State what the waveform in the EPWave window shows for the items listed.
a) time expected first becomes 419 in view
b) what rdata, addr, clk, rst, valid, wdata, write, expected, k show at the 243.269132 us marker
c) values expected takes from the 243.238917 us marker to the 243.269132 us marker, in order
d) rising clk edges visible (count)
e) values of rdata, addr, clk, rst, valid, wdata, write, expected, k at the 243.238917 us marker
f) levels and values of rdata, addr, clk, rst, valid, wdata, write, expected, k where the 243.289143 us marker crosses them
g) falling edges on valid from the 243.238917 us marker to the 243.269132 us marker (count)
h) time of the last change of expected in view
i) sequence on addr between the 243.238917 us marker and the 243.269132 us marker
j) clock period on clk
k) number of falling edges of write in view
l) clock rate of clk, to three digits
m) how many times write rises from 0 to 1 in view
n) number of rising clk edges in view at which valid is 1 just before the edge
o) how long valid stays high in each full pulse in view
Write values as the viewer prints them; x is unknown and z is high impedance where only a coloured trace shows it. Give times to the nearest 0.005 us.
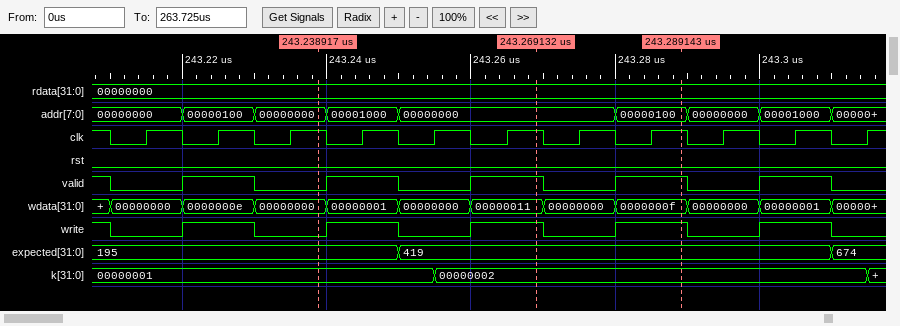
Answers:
243.25 us
rdata=00000000, addr=00000000, clk=1, rst=0, valid=1, wdata=00000011, write=1, expected=419, k=00000002
195, 419
11
rdata=00000000, addr=00000000, clk=1, rst=0, valid=0, wdata=00000000, write=0, expected=195, k=00000001
rdata=00000000, addr=00000100, clk=1, rst=0, valid=1, wdata=0000000f, write=1, expected=419, k=00000002
1
243.31 us
00000000, 00001000, 00000000
0.01 us
6
100 MHz
5
5
0.01 us, 0.01 us, 0.01 us, 0.01 us, 0.01 us
